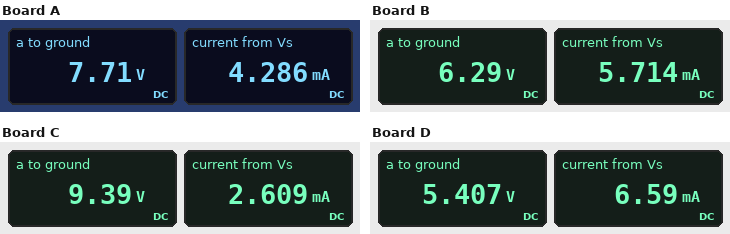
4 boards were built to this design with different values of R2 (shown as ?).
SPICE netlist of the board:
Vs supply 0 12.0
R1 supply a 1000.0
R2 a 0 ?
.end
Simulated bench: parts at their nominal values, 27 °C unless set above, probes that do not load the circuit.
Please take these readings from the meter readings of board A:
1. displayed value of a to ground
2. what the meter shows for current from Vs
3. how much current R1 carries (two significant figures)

7.71 V
4.286 mA
4.3 mA
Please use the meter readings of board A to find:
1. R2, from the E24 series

1.8 kΩ
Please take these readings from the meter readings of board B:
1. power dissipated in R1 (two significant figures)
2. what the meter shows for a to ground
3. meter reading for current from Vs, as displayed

33 mW
6.29 V
5.714 mA
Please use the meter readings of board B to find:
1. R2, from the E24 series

1.1 kΩ
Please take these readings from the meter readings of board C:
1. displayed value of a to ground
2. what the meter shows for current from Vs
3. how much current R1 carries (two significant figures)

9.39 V
2.609 mA
2.6 mA
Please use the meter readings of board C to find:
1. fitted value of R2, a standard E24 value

3.6 kΩ
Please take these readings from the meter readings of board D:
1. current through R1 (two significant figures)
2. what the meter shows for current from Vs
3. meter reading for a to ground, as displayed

6.6 mA
6.59 mA
5.407 V
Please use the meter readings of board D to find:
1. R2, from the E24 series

820 Ω
